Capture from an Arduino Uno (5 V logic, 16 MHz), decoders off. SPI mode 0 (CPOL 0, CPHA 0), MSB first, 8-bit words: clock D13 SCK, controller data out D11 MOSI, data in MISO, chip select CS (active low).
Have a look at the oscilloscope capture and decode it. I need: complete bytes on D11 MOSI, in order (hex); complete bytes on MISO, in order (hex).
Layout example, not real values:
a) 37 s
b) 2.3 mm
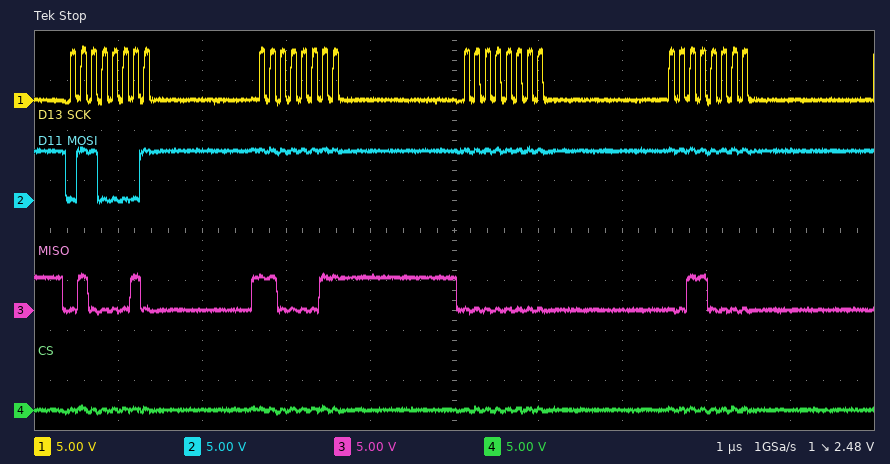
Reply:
a) 61 FF FF FF
b) 42 C3 00 30
